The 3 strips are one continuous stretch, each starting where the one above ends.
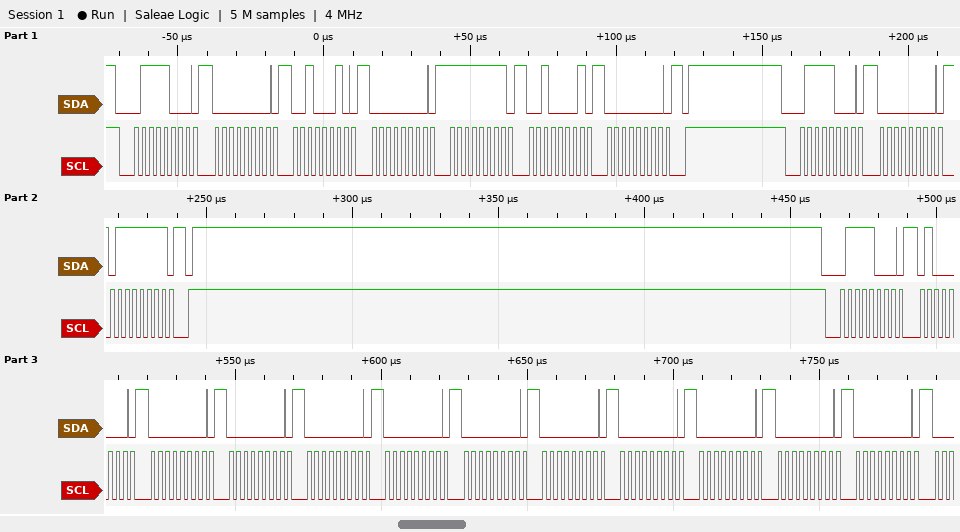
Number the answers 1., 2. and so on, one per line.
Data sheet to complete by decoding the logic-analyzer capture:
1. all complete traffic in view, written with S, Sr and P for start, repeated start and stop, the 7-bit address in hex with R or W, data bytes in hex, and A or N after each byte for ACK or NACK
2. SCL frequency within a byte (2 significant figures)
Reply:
1. S 3CW A 00 A 22 A 00 A FF A 21 A 00 A P S 3CW A 00 A 7F A P S 3CW A 40 A 00 A 00 A 00 A 00 A 00 A 00 A 00 A 00 A 00 A 00 A
2. 400 kHz
